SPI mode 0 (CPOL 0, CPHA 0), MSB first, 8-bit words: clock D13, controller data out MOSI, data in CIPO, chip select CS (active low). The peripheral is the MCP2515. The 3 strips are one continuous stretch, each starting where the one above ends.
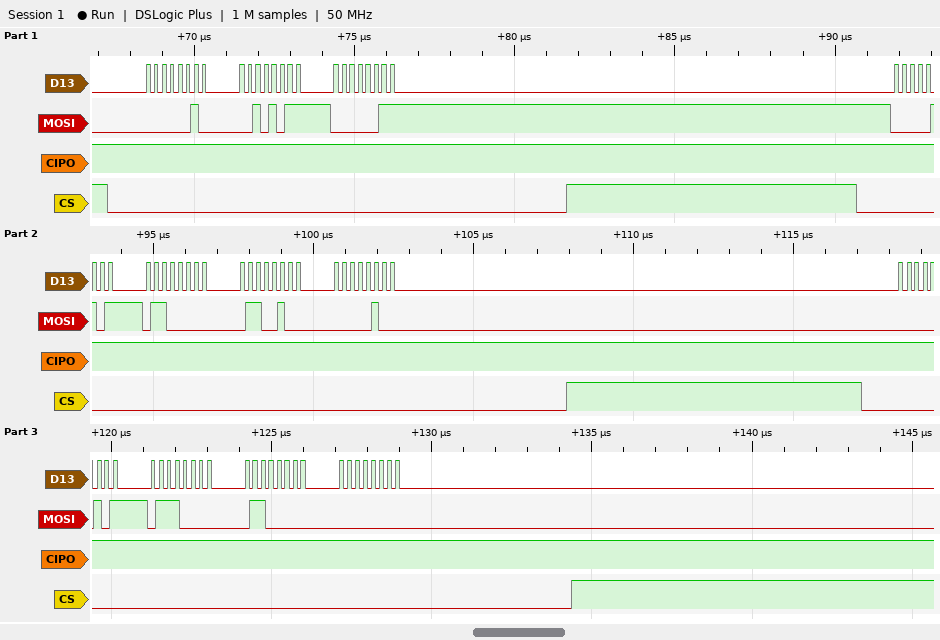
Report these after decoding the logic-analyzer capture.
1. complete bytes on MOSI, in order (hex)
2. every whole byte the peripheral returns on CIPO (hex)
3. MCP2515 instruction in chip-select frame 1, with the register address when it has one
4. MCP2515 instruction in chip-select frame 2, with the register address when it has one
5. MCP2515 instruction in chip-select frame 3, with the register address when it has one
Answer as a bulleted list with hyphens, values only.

- 02 2B 03 05 60 64 04 05 70 60 00
- FF FF FF FF FF FF FF FF FF FF FF
- WRITE 0x2B
- BIT MODIFY 0x60
- BIT MODIFY 0x70
